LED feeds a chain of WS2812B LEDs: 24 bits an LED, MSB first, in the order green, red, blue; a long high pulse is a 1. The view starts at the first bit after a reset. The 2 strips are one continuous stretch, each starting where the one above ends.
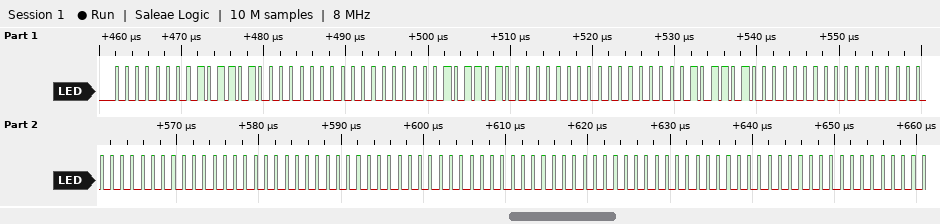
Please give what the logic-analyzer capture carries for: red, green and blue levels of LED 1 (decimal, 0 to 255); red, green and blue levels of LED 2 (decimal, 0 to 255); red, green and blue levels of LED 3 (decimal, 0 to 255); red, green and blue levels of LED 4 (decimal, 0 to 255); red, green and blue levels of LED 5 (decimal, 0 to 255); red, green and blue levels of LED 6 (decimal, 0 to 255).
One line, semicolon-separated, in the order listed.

180, 0, 0; 180, 0, 0; 180, 0, 0; 0, 0, 0; 0, 0, 0; 0, 0, 0
